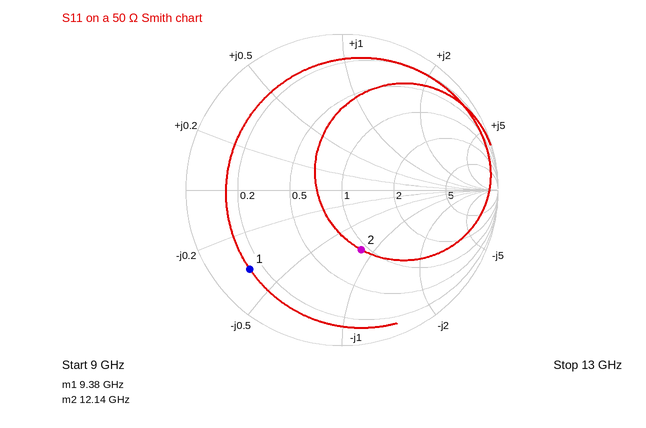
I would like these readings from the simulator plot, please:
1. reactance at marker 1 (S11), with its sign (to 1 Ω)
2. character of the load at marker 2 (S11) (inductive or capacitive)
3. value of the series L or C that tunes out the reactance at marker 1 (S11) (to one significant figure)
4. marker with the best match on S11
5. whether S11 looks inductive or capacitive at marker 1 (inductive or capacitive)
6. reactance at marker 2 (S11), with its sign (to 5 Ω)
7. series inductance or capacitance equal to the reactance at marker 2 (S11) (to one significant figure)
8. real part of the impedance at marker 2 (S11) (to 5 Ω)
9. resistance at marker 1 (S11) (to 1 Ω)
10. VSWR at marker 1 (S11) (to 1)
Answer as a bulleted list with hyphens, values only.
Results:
- -18 Ω
- capacitive
- 300 pH
- marker 2
- capacitive
- -40 Ω
- 300 fF
- 45 Ω
- 7 Ω
- 8
